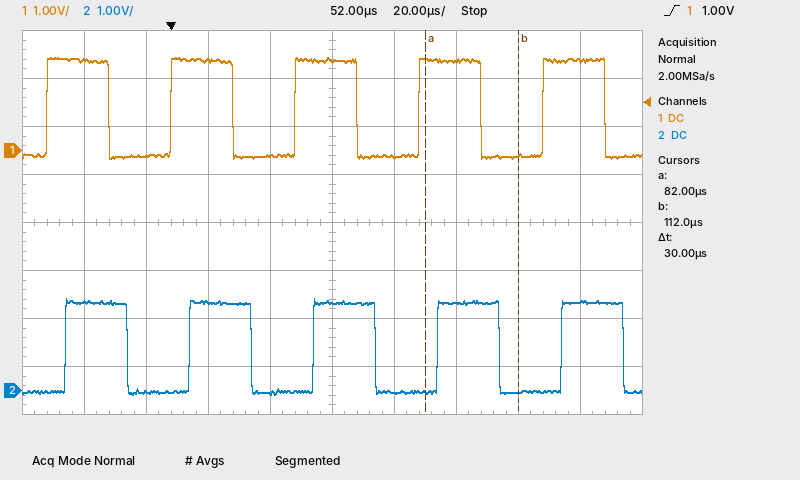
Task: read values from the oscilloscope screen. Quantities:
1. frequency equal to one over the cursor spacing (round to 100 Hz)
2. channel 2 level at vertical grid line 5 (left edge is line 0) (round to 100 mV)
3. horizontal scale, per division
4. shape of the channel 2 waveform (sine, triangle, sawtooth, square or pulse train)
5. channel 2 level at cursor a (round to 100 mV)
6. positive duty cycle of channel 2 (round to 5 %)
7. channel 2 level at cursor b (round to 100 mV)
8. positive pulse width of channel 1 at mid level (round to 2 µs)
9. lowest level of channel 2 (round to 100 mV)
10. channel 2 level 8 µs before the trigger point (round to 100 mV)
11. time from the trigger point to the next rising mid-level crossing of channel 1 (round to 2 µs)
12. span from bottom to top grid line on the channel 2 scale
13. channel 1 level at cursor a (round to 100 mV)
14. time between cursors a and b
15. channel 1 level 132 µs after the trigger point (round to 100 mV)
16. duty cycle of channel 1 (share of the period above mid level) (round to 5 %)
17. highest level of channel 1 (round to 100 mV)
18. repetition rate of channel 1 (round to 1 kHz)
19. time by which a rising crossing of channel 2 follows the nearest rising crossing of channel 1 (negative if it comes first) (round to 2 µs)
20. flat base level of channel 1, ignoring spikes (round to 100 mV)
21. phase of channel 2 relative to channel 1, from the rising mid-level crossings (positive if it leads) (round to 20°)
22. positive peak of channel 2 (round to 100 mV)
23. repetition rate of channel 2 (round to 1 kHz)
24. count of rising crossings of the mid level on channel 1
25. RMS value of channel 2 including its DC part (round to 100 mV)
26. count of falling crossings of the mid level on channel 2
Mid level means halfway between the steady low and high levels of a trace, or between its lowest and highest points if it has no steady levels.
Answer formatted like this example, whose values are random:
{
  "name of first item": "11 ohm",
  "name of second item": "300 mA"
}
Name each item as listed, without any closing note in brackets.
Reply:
{
  "frequency equal to one over the cursor spacing": "33.3 kHz",
  "channel 2 level at vertical grid line 5 (left edge is line 0)": "1.8 V",
  "horizontal scale, per division": "20 µs",
  "shape of the channel 2 waveform": "square",
  "channel 2 level at cursor a": "0.0 V",
  "positive duty cycle of channel 2": "50 %",
  "channel 2 level at cursor b": "0.0 V",
  "positive pulse width of channel 1 at mid level": "20 µs",
  "lowest level of channel 2": "-100 mV",
  "channel 2 level 8 µs before the trigger point": "0.0 V",
  "time from the trigger point to the next rising mid-level crossing of channel 1": "40 µs",
  "span from bottom to top grid line on the channel 2 scale": "8 V",
  "channel 1 level at cursor a": "1.9 V",
  "time between cursors a and b": "30 µs",
  "channel 1 level 132 µs after the trigger point": "1.9 V",
  "duty cycle of channel 1 (share of the period above mid level)": "50 %",
  "highest level of channel 1": "1.9 V",
  "repetition rate of channel 1": "25 kHz",
  "time by which a rising crossing of channel 2 follows the nearest rising crossing of channel 1 (negative if it comes first)": "+6 µs",
  "flat base level of channel 1, ignoring spikes": "-100 mV",
  "phase of channel 2 relative to channel 1, from the rising mid-level crossings (positive if it leads)": "-60°",
  "positive peak of channel 2": "1.9 V",
  "repetition rate of channel 2": "25 kHz",
  "count of rising crossings of the mid level on channel 1": "5",
  "RMS value of channel 2 including its DC part": "1.3 V",
  "count of falling crossings of the mid level on channel 2": "5"
}
